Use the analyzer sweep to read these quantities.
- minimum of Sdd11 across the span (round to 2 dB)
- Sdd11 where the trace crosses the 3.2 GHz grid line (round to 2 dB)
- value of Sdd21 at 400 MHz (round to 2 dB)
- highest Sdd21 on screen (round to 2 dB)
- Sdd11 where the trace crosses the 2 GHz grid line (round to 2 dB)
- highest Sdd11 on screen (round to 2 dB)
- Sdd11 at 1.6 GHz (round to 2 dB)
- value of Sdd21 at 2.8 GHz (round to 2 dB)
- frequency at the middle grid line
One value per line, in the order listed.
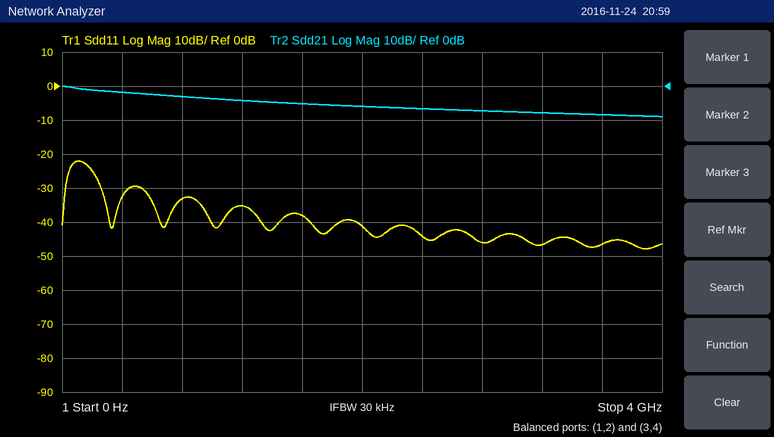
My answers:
-48 dB
-46 dB
-2 dB
0 dB
-42 dB
-22 dB
-38 dB
-8 dB
2 GHz
